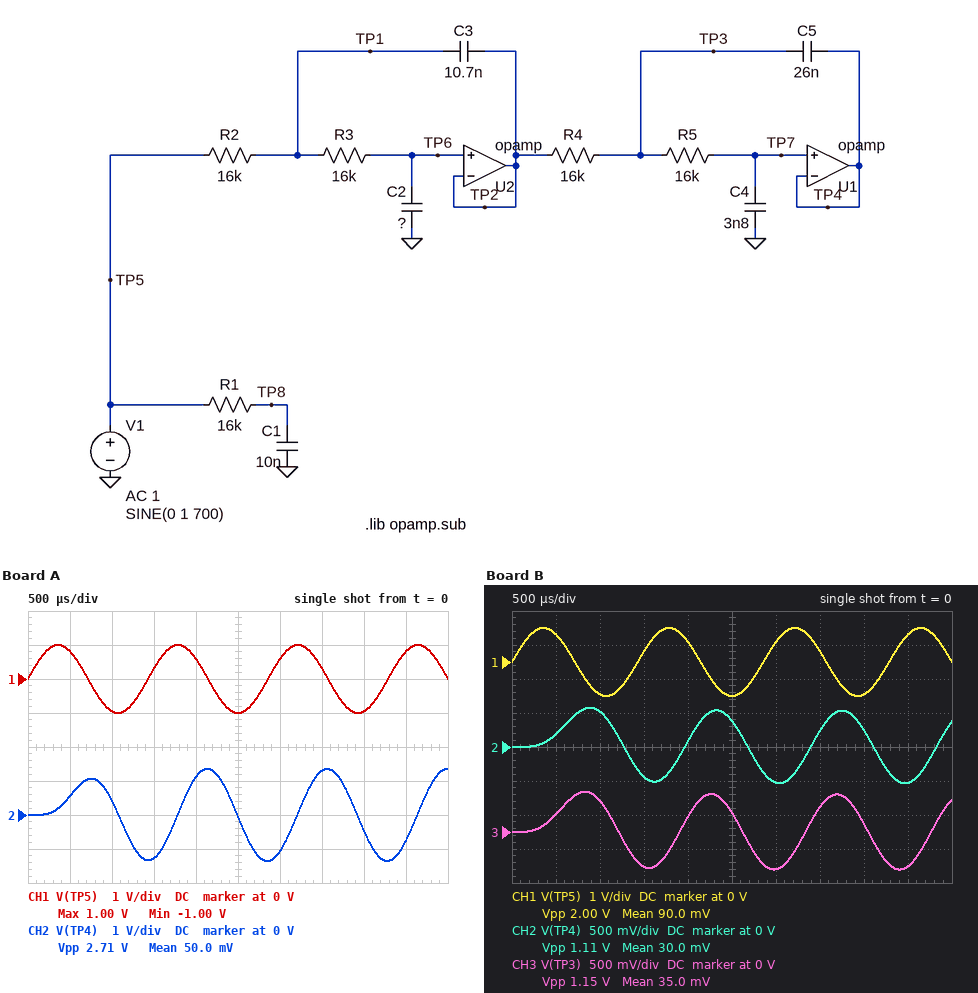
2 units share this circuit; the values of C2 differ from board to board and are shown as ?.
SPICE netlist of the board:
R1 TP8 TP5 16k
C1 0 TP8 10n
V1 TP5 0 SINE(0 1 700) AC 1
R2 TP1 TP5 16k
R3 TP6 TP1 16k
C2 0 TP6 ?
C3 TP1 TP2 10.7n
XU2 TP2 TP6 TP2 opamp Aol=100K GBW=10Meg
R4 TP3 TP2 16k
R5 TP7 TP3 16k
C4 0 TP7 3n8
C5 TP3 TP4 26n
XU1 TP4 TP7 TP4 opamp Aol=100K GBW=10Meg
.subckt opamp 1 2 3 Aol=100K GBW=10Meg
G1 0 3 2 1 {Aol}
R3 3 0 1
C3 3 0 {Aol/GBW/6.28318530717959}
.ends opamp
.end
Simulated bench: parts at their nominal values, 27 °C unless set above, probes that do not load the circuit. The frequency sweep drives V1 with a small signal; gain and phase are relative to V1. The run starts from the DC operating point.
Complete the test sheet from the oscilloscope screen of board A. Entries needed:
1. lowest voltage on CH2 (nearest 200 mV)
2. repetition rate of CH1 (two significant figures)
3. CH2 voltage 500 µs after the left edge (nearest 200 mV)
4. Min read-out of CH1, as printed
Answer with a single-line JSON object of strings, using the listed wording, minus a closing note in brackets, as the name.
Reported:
{"lowest voltage on CH2": "-1.4 V", "repetition rate of CH1": "700 Hz", "CH2 voltage 500 µs after the left edge": "600 mV", "Min read-out of CH1, as printed": "-1.00 V"}
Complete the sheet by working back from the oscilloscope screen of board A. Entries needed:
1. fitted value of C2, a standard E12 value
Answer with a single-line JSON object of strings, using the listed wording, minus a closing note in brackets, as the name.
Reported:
{"fitted value of C2, a standard E12 value": "4.7 nF"}
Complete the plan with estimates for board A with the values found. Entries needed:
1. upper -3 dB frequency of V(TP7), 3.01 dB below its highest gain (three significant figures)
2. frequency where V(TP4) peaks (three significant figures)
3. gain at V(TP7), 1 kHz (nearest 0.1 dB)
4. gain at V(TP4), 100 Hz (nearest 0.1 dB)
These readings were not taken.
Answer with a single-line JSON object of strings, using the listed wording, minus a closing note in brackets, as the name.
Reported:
{"upper -3 dB frequency of V(TP7), 3.01 dB below its highest gain": "1.13 kHz", "frequency where V(TP4) peaks": "810 Hz", "gain at V(TP7), 1 kHz": "1.8 dB", "gain at V(TP4), 100 Hz": "0.1 dB"}
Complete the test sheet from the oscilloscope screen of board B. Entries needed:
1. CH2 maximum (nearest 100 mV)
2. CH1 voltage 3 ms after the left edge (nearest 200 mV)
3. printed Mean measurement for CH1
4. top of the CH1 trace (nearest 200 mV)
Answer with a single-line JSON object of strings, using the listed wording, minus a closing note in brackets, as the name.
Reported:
{"CH2 maximum": "600 mV", "CH1 voltage 3 ms after the left edge": "600 mV", "printed Mean measurement for CH1": "90.0 mV", "top of the CH1 trace": "1.0 V"}
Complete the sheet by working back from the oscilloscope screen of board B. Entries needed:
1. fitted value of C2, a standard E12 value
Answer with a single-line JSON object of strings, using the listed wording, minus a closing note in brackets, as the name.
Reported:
{"fitted value of C2, a standard E12 value": "18 nF"}
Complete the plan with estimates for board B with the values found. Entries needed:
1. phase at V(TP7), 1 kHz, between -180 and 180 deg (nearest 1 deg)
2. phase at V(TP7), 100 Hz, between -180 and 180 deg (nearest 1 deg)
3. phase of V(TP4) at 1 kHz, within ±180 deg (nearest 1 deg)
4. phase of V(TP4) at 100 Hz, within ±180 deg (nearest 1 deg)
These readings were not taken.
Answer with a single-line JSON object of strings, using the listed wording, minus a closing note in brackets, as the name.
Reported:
{"phase at V(TP7), 1 kHz, between -180 and 180 deg": "165 deg", "phase at V(TP7), 100 Hz, between -180 and 180 deg": "-25 deg", "phase of V(TP4) at 1 kHz, within ±180 deg": "165 deg", "phase of V(TP4) at 100 Hz, within ±180 deg": "-25 deg"}
